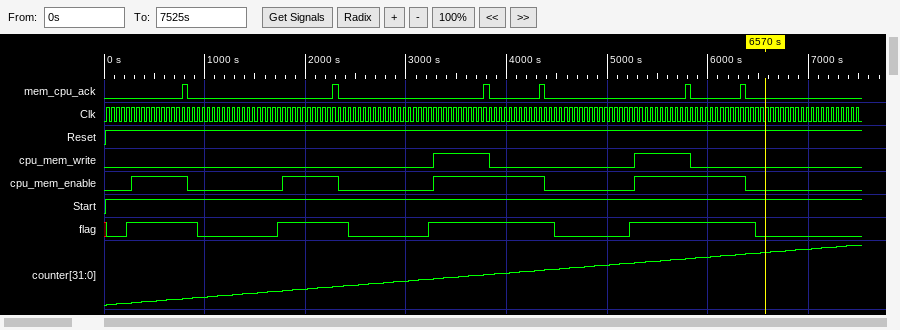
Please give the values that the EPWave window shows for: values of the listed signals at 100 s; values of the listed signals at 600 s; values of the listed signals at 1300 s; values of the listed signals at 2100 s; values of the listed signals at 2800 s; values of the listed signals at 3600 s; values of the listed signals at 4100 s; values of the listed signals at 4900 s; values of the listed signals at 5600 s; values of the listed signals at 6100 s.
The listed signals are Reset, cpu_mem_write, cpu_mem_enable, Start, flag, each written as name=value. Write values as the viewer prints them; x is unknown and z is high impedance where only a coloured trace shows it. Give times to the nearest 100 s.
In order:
Reset=1, cpu_mem_write=0, cpu_mem_enable=0, Start=1, flag=0
Reset=1, cpu_mem_write=0, cpu_mem_enable=1, Start=1, flag=1
Reset=1, cpu_mem_write=0, cpu_mem_enable=0, Start=1, flag=0
Reset=1, cpu_mem_write=0, cpu_mem_enable=1, Start=1, flag=1
Reset=1, cpu_mem_write=0, cpu_mem_enable=0, Start=1, flag=0
Reset=1, cpu_mem_write=1, cpu_mem_enable=1, Start=1, flag=1
Reset=1, cpu_mem_write=0, cpu_mem_enable=1, Start=1, flag=1
Reset=1, cpu_mem_write=0, cpu_mem_enable=0, Start=1, flag=0
Reset=1, cpu_mem_write=1, cpu_mem_enable=1, Start=1, flag=1
Reset=1, cpu_mem_write=0, cpu_mem_enable=1, Start=1, flag=1
